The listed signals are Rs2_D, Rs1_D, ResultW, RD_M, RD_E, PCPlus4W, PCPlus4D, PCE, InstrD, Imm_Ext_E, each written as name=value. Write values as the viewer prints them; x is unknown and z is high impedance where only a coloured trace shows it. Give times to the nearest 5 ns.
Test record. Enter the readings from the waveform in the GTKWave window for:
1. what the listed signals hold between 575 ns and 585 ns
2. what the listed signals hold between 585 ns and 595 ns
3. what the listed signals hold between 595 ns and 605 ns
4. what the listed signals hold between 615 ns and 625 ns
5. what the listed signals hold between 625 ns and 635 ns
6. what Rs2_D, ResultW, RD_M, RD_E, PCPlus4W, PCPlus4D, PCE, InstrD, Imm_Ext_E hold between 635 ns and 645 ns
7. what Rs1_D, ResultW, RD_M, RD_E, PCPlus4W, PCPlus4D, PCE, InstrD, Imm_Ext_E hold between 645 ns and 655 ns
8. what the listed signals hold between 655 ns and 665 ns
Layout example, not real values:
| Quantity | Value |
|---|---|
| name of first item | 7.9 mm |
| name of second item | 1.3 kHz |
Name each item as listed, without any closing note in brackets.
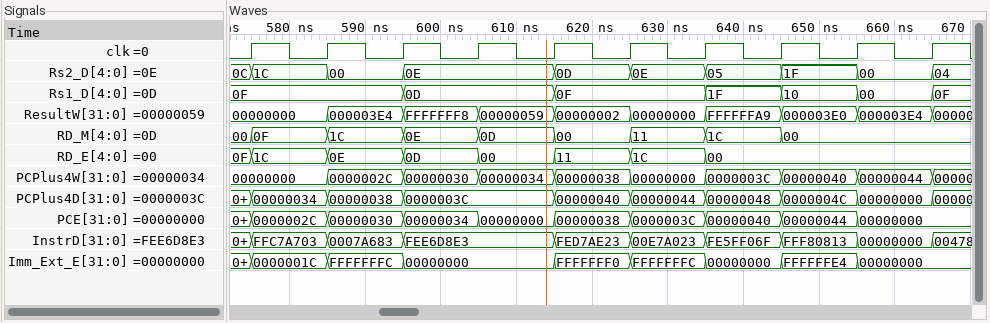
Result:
| Quantity | Value |
|---|---|
| what the listed signals hold between 575 ns and 585 ns | Rs2_D=1C, Rs1_D=0F, ResultW=00000000, RD_M=0F, RD_E=1C, PCPlus4W=00000000, PCPlus4D=00000034, PCE=0000002C, InstrD=FFC7A703, Imm_Ext_E=0000001C |
| what the listed signals hold between 585 ns and 595 ns | Rs2_D=00, Rs1_D=0F, ResultW=000003E4, RD_M=1C, RD_E=0E, PCPlus4W=0000002C, PCPlus4D=00000038, PCE=00000030, InstrD=0007A683, Imm_Ext_E=FFFFFFFC |
| what the listed signals hold between 595 ns and 605 ns | Rs2_D=0E, Rs1_D=0D, ResultW=FFFFFFF8, RD_M=0E, RD_E=0D, PCPlus4W=00000030, PCPlus4D=0000003C, PCE=00000034, InstrD=FEE6D8E3, Imm_Ext_E=00000000 |
| what the listed signals hold between 615 ns and 625 ns | Rs2_D=0D, Rs1_D=0F, ResultW=00000002, RD_M=00, RD_E=11, PCPlus4W=00000038, PCPlus4D=00000040, PCE=00000038, InstrD=FED7AE23, Imm_Ext_E=FFFFFFF0 |
| what the listed signals hold between 625 ns and 635 ns | Rs2_D=0E, Rs1_D=0F, ResultW=00000000, RD_M=11, RD_E=1C, PCPlus4W=00000000, PCPlus4D=00000044, PCE=0000003C, InstrD=00E7A023, Imm_Ext_E=FFFFFFFC |
| what Rs2_D, ResultW, RD_M, RD_E, PCPlus4W, PCPlus4D, PCE, InstrD, Imm_Ext_E hold between 635 ns and 645 ns | Rs2_D=05, ResultW=FFFFFFA9, RD_M=1C, RD_E=00, PCPlus4W=0000003C, PCPlus4D=00000048, PCE=00000040, InstrD=FE5FF06F, Imm_Ext_E=00000000 |
| what Rs1_D, ResultW, RD_M, RD_E, PCPlus4W, PCPlus4D, PCE, InstrD, Imm_Ext_E hold between 645 ns and 655 ns | Rs1_D=10, ResultW=000003E0, RD_M=00, RD_E=00, PCPlus4W=00000040, PCPlus4D=0000004C, PCE=00000044, InstrD=FFF80813, Imm_Ext_E=FFFFFFE4 |
| what the listed signals hold between 655 ns and 665 ns | Rs2_D=00, Rs1_D=00, ResultW=000003E4, RD_M=00, RD_E=00, PCPlus4W=00000044, PCPlus4D=00000000, PCE=00000000, InstrD=00000000, Imm_Ext_E=00000000 |
